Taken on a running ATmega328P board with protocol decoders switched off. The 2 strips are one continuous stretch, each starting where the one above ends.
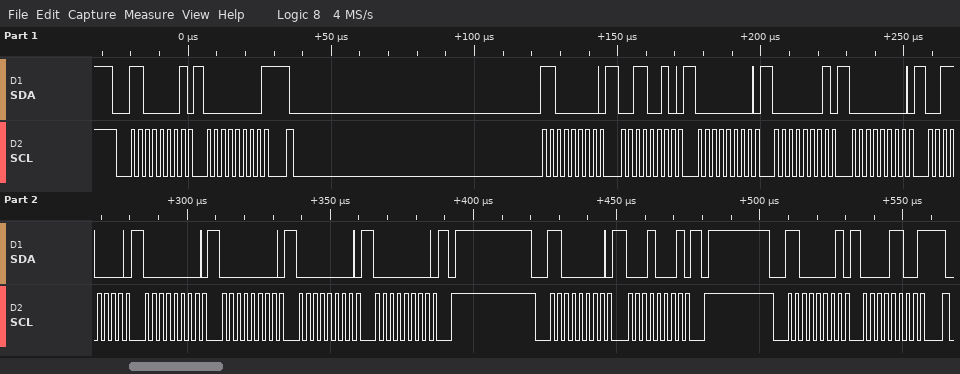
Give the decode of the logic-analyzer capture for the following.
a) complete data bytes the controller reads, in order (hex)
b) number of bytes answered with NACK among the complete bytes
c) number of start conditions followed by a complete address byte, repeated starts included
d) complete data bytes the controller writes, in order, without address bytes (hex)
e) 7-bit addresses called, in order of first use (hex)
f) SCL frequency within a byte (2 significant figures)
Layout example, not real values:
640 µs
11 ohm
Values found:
00 0C
2
4
32 00 01 00 30 00 00 00 00 11
0x60
400 kHz
